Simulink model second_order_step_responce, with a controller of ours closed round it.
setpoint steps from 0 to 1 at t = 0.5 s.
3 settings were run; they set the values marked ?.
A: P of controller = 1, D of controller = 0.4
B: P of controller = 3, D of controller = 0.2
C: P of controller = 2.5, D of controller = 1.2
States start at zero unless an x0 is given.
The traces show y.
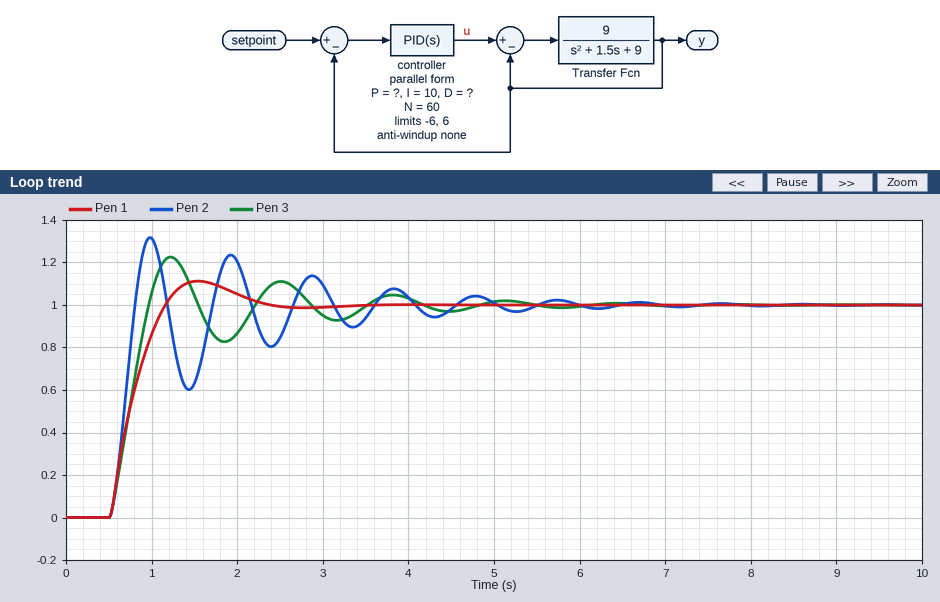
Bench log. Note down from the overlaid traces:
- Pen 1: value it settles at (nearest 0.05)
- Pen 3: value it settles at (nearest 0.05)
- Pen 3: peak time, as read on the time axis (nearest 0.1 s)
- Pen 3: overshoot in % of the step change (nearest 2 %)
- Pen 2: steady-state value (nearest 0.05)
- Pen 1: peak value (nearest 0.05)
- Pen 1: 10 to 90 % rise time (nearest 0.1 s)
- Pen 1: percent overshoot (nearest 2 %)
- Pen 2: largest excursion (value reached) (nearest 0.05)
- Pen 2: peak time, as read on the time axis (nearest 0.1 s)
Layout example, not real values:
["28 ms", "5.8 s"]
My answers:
["1.00", "1.00", "1.2 s", "22 %", "1.00", "1.10", "0.5 s", "12 %", "1.30", "1.0 s"]
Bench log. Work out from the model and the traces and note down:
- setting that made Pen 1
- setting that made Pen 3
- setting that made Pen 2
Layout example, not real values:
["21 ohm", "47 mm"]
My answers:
["C", "A", "B"]
